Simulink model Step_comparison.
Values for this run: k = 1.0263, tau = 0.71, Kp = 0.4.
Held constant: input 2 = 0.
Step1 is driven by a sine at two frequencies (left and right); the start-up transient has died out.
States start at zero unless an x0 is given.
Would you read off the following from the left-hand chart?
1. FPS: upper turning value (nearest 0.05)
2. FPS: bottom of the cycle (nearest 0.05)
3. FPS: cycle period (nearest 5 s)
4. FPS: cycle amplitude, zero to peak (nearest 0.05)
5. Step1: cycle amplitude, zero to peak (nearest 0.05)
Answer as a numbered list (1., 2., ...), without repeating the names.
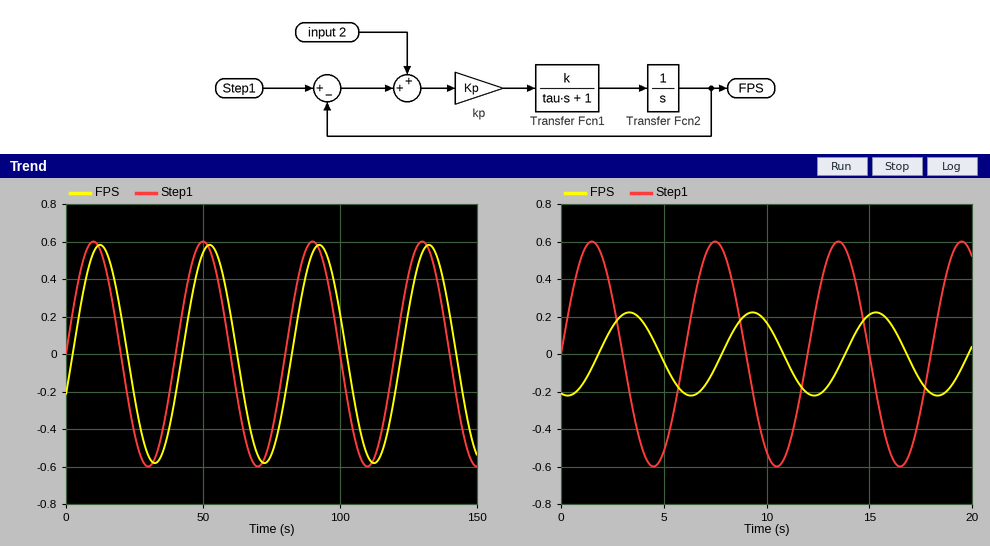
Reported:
1. 0.60
2. -0.60
3. 40 s
4. 0.60
5. 0.60
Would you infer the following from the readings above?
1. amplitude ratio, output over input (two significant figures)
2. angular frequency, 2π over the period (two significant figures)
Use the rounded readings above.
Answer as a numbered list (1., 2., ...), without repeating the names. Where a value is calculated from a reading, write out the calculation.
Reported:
1. 0.6 / 0.6 = 1.0
2. 2π / 40 = 0.16 rad/s
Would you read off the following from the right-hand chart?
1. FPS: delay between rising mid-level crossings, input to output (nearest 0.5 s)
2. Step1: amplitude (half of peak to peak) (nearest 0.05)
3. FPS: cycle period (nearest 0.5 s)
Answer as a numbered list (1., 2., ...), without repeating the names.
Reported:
1. 2.0 s
2. 0.60
3. 6.0 s
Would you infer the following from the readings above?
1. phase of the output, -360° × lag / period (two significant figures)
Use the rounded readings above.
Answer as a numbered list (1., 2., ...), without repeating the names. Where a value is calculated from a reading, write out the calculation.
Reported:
1. -360 × 2 / 6 = -120°
